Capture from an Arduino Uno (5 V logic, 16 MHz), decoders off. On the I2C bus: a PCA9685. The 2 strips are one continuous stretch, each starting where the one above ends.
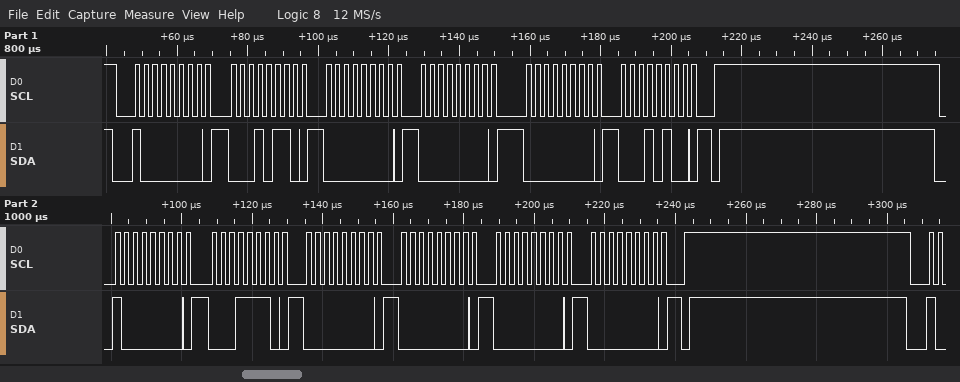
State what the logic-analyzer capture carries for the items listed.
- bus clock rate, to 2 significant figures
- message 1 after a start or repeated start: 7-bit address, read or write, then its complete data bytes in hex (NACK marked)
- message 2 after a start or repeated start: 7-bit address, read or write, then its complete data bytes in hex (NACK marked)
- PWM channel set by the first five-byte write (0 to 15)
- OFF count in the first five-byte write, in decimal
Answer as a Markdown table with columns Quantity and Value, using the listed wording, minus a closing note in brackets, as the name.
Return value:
| Quantity | Value |
|---|---|
| bus clock rate, to 2 significant figures | 400 kHz |
| message 1 after a start or repeated start: 7-bit address, read or write, then its complete data bytes in hex | 0x40 write: 16 00 00 00 14 |
| message 2 after a start or repeated start: 7-bit address, read or write, then its complete data bytes in hex | 0x40 write: 1E 00 00 00 00 |
| PWM channel set by the first five-byte write | 4 |
| OFF count in the first five-byte write, in decimal | 5120 |
